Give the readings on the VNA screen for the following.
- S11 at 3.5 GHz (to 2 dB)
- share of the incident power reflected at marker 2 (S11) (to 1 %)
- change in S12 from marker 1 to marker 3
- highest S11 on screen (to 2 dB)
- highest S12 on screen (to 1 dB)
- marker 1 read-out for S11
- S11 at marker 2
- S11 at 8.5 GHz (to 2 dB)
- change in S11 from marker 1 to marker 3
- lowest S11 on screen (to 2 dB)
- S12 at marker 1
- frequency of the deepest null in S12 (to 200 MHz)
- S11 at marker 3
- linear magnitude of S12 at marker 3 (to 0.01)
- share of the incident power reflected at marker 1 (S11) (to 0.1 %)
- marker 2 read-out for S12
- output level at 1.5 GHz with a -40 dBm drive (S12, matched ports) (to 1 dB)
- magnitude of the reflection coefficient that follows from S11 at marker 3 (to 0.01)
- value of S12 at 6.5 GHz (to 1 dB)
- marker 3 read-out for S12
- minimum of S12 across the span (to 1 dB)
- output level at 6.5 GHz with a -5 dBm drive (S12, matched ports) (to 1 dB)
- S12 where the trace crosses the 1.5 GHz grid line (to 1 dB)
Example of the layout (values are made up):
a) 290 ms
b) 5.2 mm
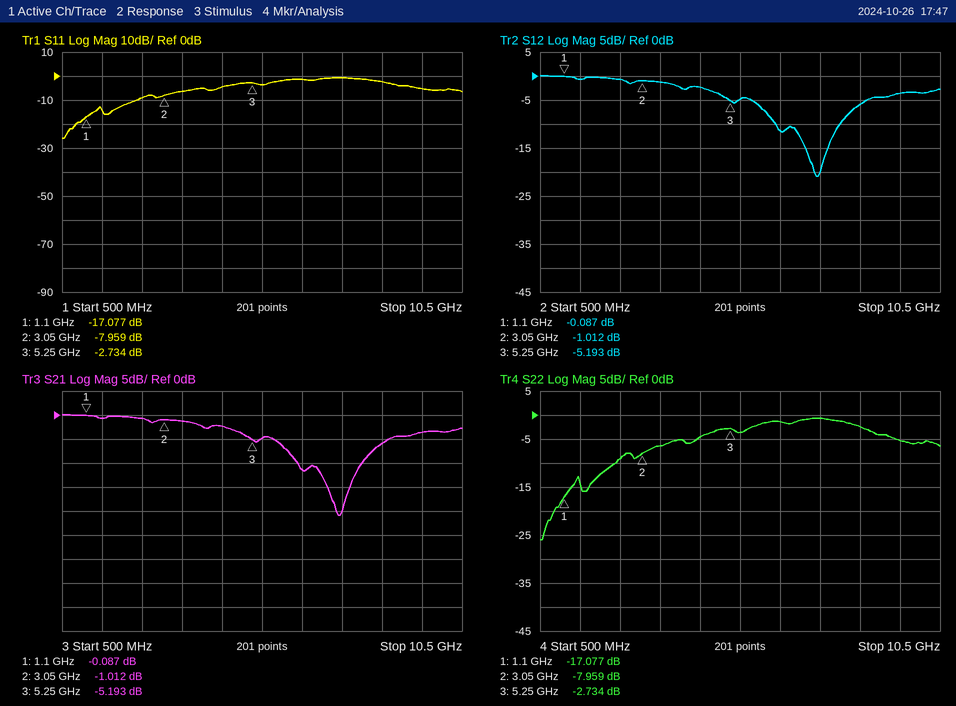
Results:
a) -6 dB
b) 16 %
c) -5.106 dB
d) 0 dB
e) 0 dB
f) -17.077 dB
g) -7.959 dB
h) -2 dB
i) 14.343 dB
j) -26 dB
k) -0.087 dB
l) 7.4 GHz
m) -2.734 dB
n) 0.55
o) 2.0 %
p) -1.012 dB
q) -41 dBm
r) 0.73
s) -11 dB
t) -5.193 dB
u) -21 dB
v) -16 dBm
w) -1 dB
